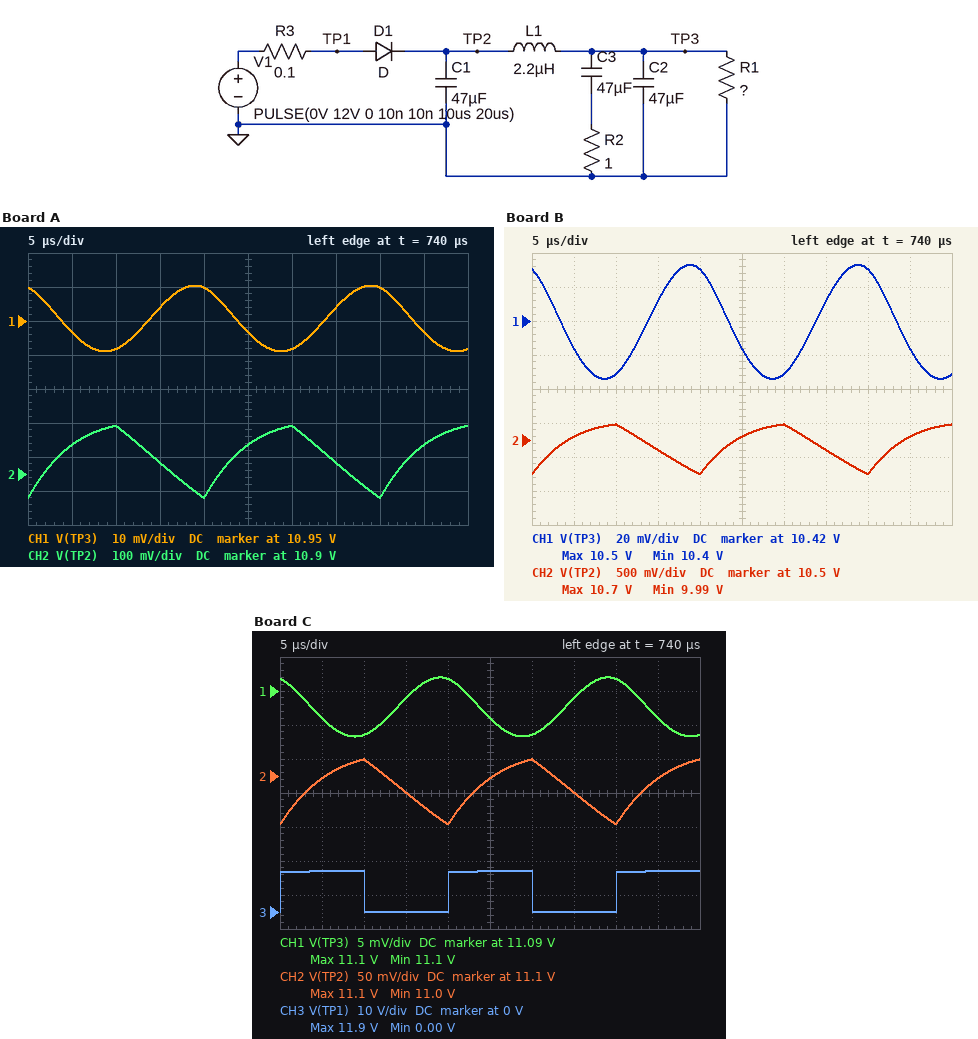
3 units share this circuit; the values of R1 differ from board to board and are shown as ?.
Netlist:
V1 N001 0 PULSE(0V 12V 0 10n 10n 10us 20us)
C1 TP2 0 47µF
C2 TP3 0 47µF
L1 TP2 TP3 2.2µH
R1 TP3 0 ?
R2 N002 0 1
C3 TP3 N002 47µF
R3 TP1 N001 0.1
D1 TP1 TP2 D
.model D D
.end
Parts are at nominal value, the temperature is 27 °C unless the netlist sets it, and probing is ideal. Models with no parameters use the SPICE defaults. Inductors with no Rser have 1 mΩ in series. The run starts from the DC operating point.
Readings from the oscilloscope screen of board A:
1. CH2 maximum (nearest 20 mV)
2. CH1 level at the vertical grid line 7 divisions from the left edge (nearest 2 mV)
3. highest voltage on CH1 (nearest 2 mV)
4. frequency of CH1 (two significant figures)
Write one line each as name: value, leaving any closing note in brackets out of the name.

CH2 maximum: 11.04 V
CH1 level at the vertical grid line 7 divisions from the left edge: 10.954 V
highest voltage on CH1: 10.960 V
frequency of CH1: 50 kHz
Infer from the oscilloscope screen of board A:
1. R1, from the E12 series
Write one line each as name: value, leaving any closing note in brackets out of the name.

R1, from the E12 series: 12 Ω
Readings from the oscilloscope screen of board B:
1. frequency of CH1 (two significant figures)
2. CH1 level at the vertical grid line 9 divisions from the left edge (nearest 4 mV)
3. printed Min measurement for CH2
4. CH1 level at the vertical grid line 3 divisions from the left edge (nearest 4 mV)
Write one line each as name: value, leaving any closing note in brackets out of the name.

frequency of CH1: 50 kHz
CH1 level at the vertical grid line 9 divisions from the left edge: 10.404 V
printed Min measurement for CH2: 9.99 V
CH1 level at the vertical grid line 3 divisions from the left edge: 10.432 V
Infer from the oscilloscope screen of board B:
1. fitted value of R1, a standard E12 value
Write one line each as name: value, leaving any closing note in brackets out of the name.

fitted value of R1, a standard E12 value: 3.3 Ω
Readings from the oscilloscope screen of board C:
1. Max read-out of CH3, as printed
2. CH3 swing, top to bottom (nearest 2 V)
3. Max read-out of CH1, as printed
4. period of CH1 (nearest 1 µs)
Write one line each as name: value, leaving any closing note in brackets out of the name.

Max read-out of CH3, as printed: 11.9 V
CH3 swing, top to bottom: 12 V
Max read-out of CH1, as printed: 11.1 V
period of CH1: 20 µs
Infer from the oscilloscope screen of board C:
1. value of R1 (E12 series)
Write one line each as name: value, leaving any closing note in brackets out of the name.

value of R1: 27 Ω
